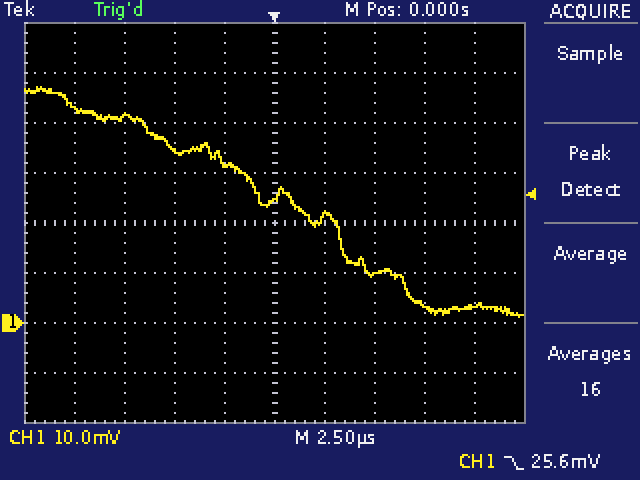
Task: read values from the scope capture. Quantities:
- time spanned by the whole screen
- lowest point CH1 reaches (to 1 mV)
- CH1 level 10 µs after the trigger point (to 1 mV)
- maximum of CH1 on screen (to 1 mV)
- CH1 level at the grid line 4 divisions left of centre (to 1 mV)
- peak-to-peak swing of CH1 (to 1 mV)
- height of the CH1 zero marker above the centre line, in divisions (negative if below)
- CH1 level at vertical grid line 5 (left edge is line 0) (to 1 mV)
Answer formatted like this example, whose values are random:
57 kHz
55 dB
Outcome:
25 µs
1 mV
3 mV
47 mV
43 mV
46 mV
-2.0 div
25 mV
